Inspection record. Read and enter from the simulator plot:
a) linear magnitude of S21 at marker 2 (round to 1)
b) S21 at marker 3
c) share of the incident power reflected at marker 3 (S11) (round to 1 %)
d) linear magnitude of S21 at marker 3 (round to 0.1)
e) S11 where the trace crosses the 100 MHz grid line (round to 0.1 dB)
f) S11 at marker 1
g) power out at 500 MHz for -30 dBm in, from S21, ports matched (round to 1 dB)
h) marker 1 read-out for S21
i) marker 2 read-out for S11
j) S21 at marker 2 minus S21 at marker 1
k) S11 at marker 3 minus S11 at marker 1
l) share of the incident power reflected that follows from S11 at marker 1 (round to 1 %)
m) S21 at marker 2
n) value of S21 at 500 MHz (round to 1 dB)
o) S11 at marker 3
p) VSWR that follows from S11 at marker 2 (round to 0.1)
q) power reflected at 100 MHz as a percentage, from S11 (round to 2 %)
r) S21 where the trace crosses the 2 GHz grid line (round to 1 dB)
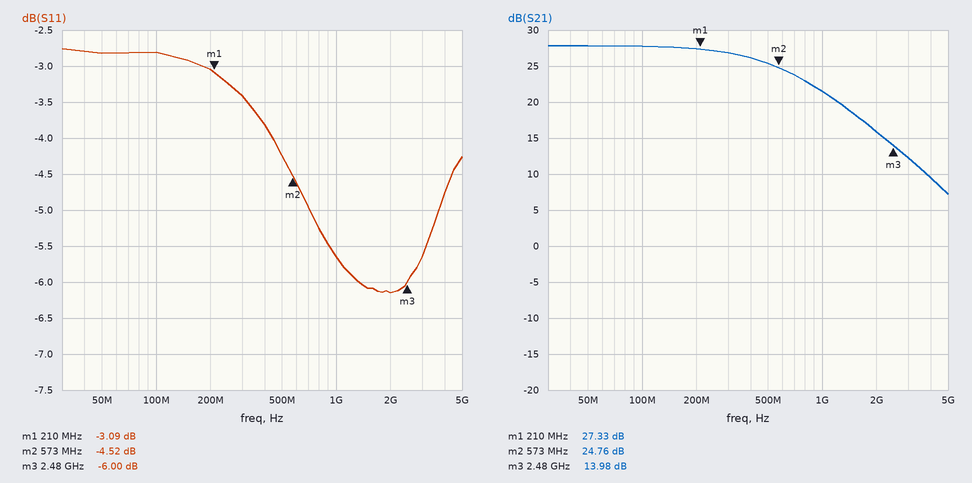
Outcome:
17
13.98 dB
25 %
5.0
-2.8 dB
-3.09 dB
-5 dBm
27.33 dB
-4.52 dB
-2.57 dB
-2.91 dB
49 %
24.76 dB
25 dB
-6.00 dB
3.9
52 %
16 dB
